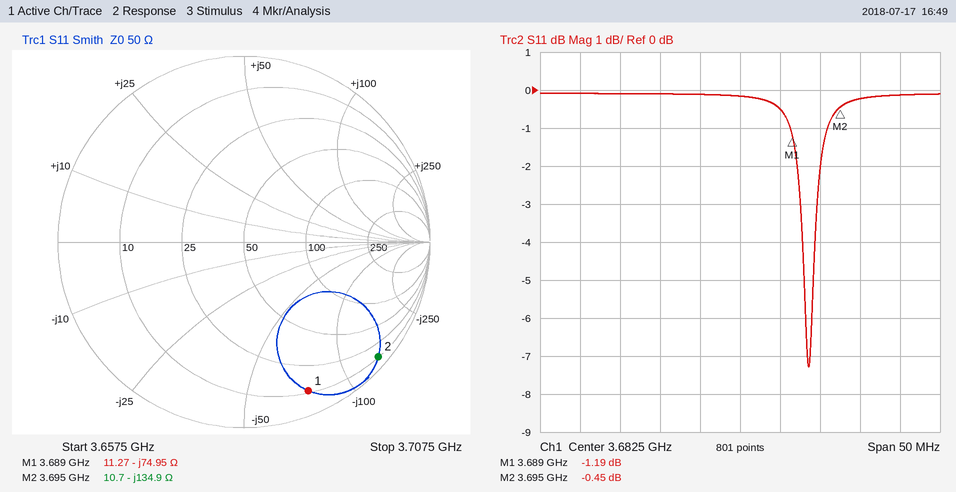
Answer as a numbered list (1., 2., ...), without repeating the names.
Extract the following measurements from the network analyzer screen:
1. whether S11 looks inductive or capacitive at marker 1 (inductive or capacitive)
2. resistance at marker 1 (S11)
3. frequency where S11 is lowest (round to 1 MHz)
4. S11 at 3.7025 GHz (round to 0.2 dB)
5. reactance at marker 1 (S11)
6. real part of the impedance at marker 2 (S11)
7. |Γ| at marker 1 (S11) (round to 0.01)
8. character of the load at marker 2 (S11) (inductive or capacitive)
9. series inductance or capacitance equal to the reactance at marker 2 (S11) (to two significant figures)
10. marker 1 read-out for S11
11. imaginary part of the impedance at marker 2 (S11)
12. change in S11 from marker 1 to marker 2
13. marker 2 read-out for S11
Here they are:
1. capacitive
2. 11.27 Ω
3. 3.691 GHz
4. -0.2 dB
5. -74.95 Ω
6. 10.7 Ω
7. 0.87
8. capacitive
9. 320 fF
10. -1.19 dB
11. -134.9 Ω
12. 0.74 dB
13. -0.45 dB
